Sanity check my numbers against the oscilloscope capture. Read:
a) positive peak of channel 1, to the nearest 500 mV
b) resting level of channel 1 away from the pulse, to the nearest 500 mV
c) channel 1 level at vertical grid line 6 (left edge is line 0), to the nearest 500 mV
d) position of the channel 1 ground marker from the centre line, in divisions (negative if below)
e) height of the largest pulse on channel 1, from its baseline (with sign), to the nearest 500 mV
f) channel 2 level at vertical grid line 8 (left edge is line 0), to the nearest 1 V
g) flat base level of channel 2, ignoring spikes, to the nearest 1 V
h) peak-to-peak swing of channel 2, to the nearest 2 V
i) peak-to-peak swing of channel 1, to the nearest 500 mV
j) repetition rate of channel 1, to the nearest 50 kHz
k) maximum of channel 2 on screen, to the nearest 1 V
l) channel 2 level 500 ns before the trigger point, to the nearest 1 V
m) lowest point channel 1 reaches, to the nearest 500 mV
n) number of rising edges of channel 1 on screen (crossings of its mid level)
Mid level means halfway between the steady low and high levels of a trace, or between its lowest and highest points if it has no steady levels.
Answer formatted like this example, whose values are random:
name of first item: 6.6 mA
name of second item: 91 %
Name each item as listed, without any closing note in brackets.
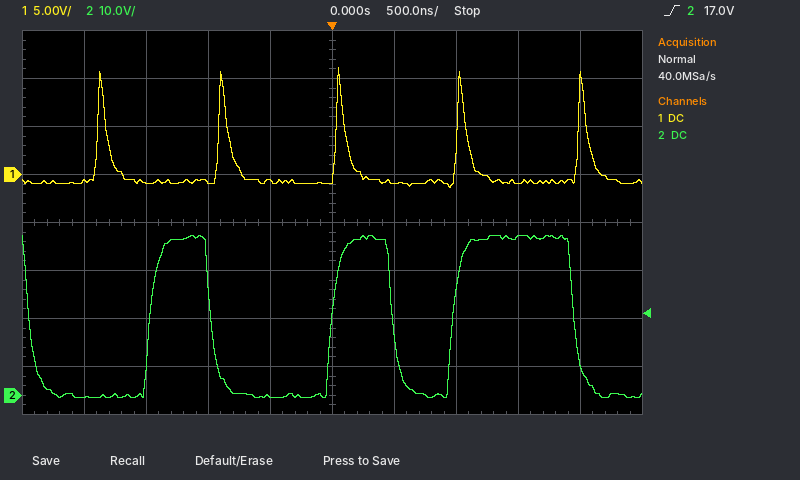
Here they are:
positive peak of channel 1, to the nearest 500 mV: 11.0 V
resting level of channel 1 away from the pulse, to the nearest 500 mV: -1.0 V
channel 1 level at vertical grid line 6 (left edge is line 0), to the nearest 500 mV: -1.0 V
position of the channel 1 ground marker from the centre line, in divisions: +1.0 div
height of the largest pulse on channel 1, from its baseline (with sign), to the nearest 500 mV: +12.0 V
channel 2 level at vertical grid line 8 (left edge is line 0), to the nearest 1 V: 33 V
flat base level of channel 2, ignoring spikes, to the nearest 1 V: 0 V
peak-to-peak swing of channel 2, to the nearest 2 V: 34 V
peak-to-peak swing of channel 1, to the nearest 500 mV: 12.5 V
repetition rate of channel 1, to the nearest 50 kHz: 1.05 MHz
maximum of channel 2 on screen, to the nearest 1 V: 33 V
channel 2 level 500 ns before the trigger point, to the nearest 1 V: 0 V
lowest point channel 1 reaches, to the nearest 500 mV: -1.5 V
number of rising edges of channel 1 on screen: 5
